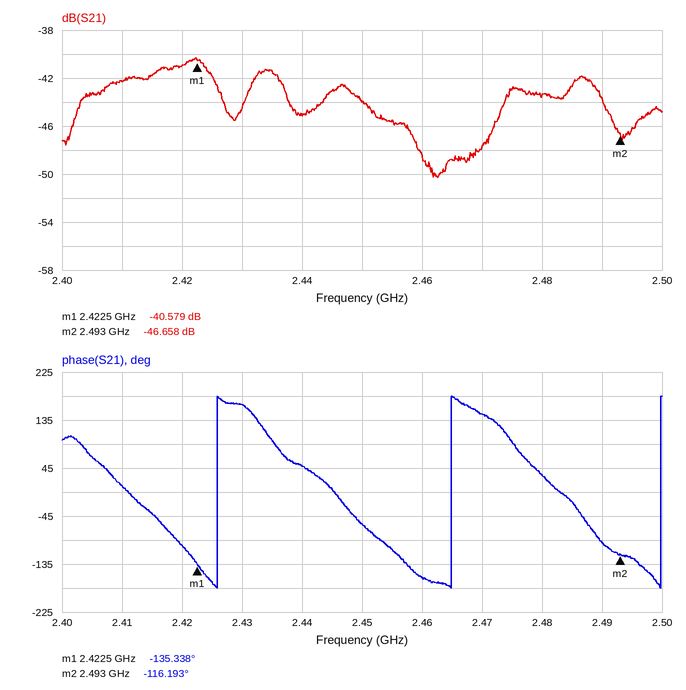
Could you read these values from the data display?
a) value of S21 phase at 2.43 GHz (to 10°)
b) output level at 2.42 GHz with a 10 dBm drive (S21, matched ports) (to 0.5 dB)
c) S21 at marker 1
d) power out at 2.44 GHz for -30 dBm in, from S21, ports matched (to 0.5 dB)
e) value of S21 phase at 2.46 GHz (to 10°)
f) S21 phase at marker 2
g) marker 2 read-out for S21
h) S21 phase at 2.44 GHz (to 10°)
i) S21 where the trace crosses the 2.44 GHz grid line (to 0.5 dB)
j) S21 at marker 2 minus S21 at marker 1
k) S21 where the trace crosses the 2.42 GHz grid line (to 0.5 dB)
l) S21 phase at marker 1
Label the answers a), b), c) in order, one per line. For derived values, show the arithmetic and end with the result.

a) 160°
b) 10 dBm + (-41.0 dB) = -31.0 dBm
c) -40.579 dB
d) -30 dBm + (-45.0 dB) = -75.0 dBm
e) -160°
f) -116.193°
g) -46.658 dB
h) 50°
i) -45.0 dB
j) -46.658 − (-40.579) = -6.079 dB
k) -41.0 dB
l) -135.338°
